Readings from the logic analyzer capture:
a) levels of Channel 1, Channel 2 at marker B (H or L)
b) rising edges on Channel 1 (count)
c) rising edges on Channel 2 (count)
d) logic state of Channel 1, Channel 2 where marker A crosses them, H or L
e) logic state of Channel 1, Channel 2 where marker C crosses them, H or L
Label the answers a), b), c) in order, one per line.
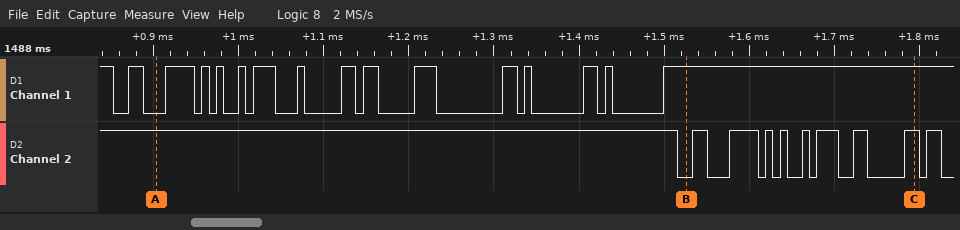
a) Channel 1=H, Channel 2=L
b) 15
c) 9
d) Channel 1=L, Channel 2=H
e) Channel 1=H, Channel 2=H
